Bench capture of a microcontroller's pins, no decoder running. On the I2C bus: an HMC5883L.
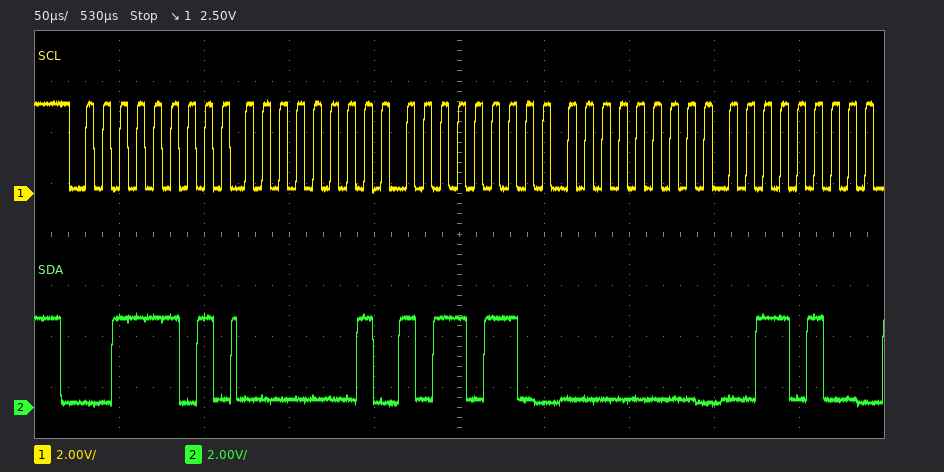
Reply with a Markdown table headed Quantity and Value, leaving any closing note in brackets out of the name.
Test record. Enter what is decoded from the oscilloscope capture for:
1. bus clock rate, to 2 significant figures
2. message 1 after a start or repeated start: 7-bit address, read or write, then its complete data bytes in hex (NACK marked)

| Quantity | Value |
|---|---|
| bus clock rate, to 2 significant figures | 100 kHz |
| message 1 after a start or repeated start: 7-bit address, read or write, then its complete data bytes in hex | 0x1E read: 01 B6 00 34 |
